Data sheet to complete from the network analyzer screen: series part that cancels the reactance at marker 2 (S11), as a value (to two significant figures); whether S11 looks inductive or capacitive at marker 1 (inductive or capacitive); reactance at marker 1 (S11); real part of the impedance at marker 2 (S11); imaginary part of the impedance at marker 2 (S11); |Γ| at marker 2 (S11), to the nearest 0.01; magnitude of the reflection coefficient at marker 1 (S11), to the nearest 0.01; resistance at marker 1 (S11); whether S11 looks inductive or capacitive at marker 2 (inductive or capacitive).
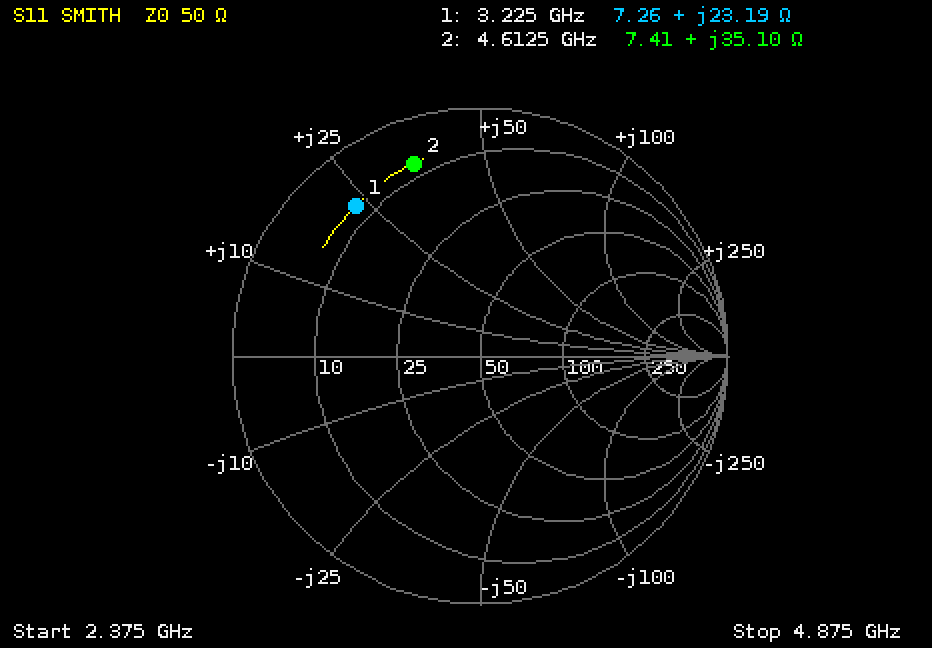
980 fF
inductive
+23.19 Ω
7.41 Ω
+35.10 Ω
0.82
0.79
7.26 Ω
inductive
